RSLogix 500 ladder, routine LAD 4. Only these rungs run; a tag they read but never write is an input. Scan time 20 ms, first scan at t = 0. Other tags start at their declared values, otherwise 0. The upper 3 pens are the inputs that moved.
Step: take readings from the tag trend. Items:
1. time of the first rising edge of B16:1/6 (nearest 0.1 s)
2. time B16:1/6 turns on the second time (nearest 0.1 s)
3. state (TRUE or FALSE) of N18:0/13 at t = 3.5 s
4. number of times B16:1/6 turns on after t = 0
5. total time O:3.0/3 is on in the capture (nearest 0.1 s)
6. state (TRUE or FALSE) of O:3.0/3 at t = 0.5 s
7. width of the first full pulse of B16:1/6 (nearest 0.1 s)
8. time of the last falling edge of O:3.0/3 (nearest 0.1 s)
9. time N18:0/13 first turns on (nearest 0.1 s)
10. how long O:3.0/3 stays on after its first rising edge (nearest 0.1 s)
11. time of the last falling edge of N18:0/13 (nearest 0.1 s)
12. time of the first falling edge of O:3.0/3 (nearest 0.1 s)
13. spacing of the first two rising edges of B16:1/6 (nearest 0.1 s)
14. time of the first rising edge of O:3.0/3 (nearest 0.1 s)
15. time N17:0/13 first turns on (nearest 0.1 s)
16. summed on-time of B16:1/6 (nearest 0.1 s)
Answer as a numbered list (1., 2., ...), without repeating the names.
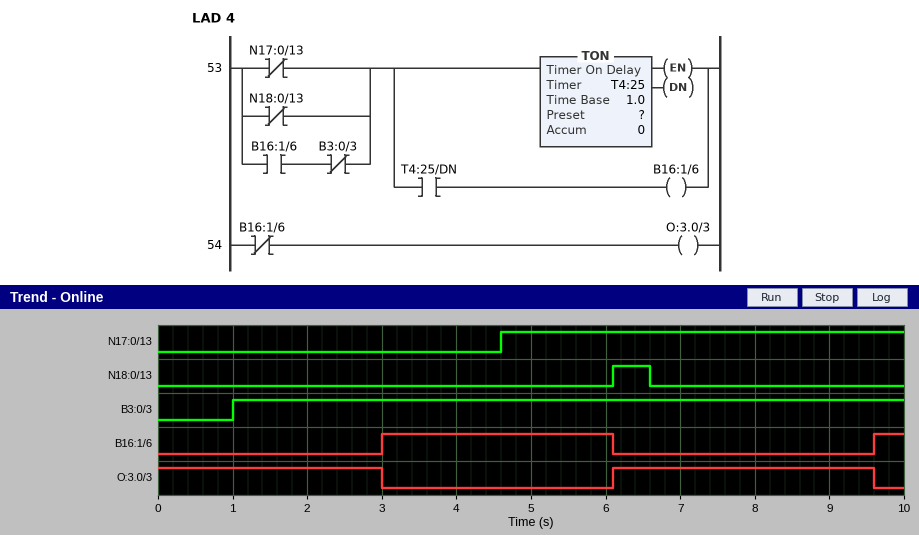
1. 3.0 s
2. 9.6 s
3. FALSE
4. 2
5. 6.5 s
6. TRUE
7. 3.1 s
8. 9.6 s
9. 6.1 s
10. 3.5 s
11. 6.6 s
12. 3.0 s
13. 6.6 s
14. 6.1 s
15. 4.6 s
16. 3.5 s
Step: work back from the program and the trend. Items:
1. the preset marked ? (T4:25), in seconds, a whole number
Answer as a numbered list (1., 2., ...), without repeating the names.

1. 3 s
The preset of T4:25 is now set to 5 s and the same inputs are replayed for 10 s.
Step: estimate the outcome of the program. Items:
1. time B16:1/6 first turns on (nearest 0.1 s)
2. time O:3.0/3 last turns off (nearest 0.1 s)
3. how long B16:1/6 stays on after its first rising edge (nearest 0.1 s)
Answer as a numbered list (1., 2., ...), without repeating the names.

1. 5.0 s
2. 5.0 s
3. 1.1 s
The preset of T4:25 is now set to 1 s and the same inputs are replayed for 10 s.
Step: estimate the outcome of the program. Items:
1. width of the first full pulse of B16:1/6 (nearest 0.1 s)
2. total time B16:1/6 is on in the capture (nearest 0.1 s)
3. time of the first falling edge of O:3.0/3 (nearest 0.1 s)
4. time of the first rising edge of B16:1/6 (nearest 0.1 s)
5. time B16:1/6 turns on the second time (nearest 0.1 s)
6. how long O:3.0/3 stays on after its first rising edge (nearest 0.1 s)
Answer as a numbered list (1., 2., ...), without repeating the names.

1. 5.1 s
2. 7.5 s
3. 1.0 s
4. 1.0 s
5. 7.6 s
6. 1.5 s
